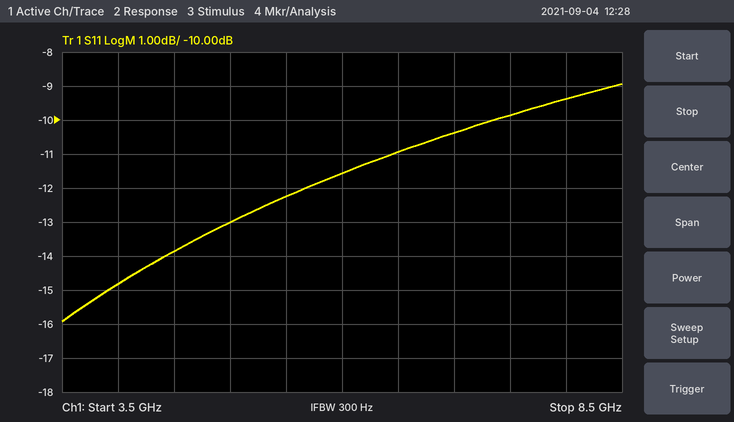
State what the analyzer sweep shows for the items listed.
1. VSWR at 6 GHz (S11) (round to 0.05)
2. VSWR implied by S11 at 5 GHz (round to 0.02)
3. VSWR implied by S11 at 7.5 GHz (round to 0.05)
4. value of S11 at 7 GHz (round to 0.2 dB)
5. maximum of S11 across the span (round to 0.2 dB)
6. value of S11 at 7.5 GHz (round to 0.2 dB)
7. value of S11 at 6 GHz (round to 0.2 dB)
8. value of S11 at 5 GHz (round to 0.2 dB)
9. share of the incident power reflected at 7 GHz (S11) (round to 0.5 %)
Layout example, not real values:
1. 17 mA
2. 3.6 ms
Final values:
1. 1.70
2. 1.58
3. 1.95
4. -10.4 dB
5. -9.0 dB
6. -9.8 dB
7. -11.6 dB
8. -13.0 dB
9. 9.0 %
